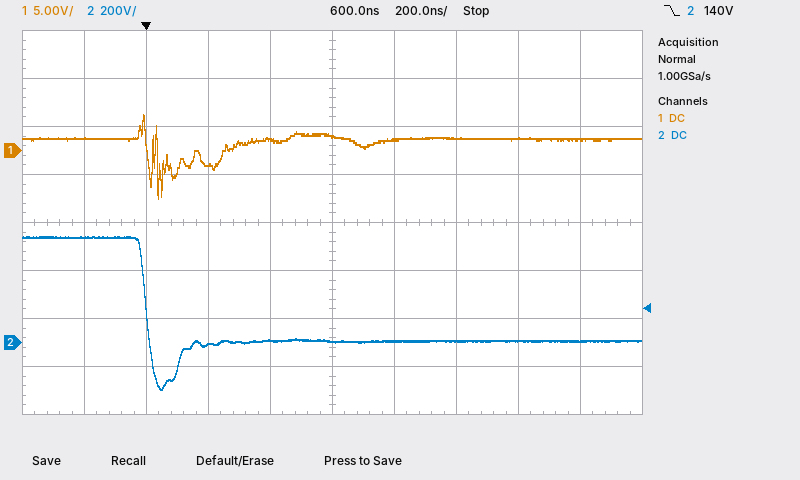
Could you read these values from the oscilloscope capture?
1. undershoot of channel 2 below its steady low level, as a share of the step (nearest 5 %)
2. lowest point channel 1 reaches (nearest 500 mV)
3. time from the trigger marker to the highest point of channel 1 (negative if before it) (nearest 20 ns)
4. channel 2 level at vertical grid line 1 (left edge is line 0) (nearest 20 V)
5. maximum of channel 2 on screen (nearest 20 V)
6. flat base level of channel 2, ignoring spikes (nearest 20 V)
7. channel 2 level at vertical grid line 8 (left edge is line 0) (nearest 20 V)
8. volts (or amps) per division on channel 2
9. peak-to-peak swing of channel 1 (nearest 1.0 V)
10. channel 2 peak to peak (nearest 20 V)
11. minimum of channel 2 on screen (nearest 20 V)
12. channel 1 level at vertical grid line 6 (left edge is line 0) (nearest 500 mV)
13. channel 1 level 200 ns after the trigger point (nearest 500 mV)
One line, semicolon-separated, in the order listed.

45 %; -5.0 V; 0 ns; 440 V; 440 V; 0 V; 0 V; 200 V; 9.0 V; 640 V; -200 V; 1.0 V; -1.5 V
